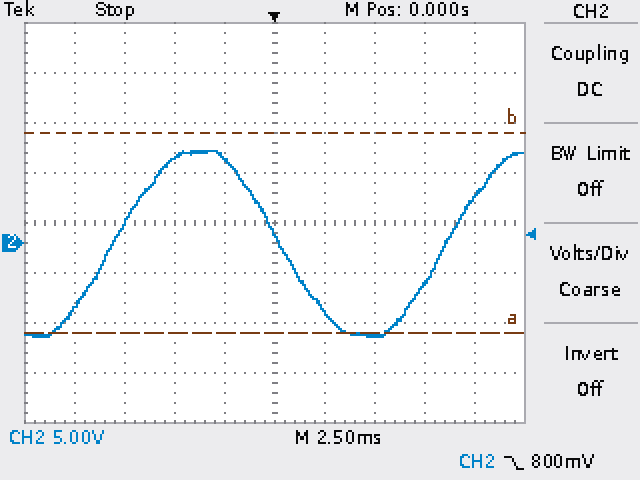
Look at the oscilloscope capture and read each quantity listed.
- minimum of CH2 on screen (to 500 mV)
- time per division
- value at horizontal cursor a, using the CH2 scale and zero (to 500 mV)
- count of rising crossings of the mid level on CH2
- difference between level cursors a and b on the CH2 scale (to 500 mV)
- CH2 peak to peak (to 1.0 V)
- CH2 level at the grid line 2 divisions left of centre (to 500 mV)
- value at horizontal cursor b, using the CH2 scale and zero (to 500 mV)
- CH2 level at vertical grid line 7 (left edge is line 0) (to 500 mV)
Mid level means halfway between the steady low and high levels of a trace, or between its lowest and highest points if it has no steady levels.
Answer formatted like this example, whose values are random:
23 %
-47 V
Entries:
-9.5 V
2.5 ms
-9.0 V
2
20.0 V
19.0 V
8.5 V
11.0 V
-9.5 V
